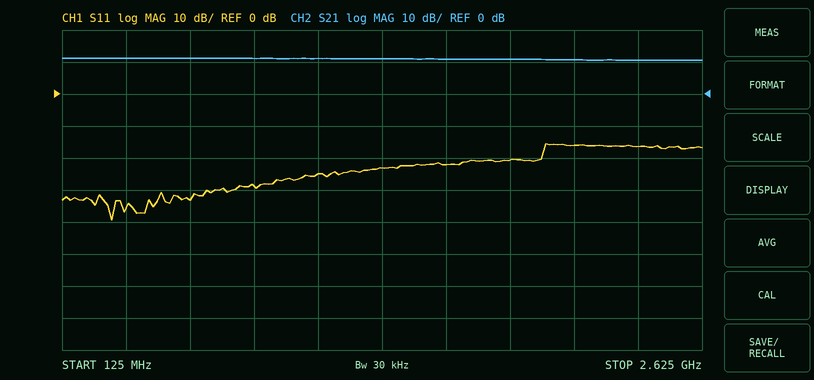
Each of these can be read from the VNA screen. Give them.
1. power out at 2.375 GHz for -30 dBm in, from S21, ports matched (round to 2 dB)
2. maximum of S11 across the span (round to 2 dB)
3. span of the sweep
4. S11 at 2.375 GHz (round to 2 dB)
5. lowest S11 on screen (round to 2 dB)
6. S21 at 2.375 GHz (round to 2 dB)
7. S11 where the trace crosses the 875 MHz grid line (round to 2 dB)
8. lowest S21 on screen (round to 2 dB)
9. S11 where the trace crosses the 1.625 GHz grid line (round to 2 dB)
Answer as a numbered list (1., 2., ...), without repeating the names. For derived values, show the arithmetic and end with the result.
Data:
1. -30 dBm + (10 dB) = -20 dBm
2. -16 dB
3. 2.5 GHz
4. -16 dB
5. -40 dB
6. 10 dB
7. -28 dB
8. 10 dB
9. -22 dB
